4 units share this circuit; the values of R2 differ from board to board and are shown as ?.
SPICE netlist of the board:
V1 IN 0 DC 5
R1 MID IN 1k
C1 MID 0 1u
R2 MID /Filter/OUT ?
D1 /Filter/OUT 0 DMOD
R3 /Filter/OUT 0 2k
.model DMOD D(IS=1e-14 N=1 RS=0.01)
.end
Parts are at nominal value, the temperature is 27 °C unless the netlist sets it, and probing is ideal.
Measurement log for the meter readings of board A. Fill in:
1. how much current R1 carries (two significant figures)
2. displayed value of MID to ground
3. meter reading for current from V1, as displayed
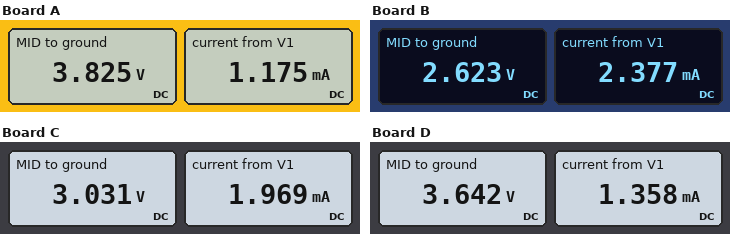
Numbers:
1.2 mA
3.825 V
1.175 mA
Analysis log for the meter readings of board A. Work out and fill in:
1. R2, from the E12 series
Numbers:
2.7 kΩ
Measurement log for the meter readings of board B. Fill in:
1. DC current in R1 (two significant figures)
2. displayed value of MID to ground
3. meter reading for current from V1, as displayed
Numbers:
2.4 mA
2.623 V
2.377 mA
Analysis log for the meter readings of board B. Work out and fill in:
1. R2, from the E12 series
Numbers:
820 Ω
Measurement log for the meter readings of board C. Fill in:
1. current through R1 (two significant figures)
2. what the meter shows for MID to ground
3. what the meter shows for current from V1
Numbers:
2.0 mA
3.031 V
1.969 mA
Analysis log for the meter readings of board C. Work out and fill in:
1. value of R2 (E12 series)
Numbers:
1.2 kΩ
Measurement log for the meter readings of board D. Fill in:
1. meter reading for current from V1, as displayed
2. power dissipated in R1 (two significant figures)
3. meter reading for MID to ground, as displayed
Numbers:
1.358 mA
1.8 mW
3.642 V
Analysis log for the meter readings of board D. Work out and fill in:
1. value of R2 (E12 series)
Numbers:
2.2 kΩ
